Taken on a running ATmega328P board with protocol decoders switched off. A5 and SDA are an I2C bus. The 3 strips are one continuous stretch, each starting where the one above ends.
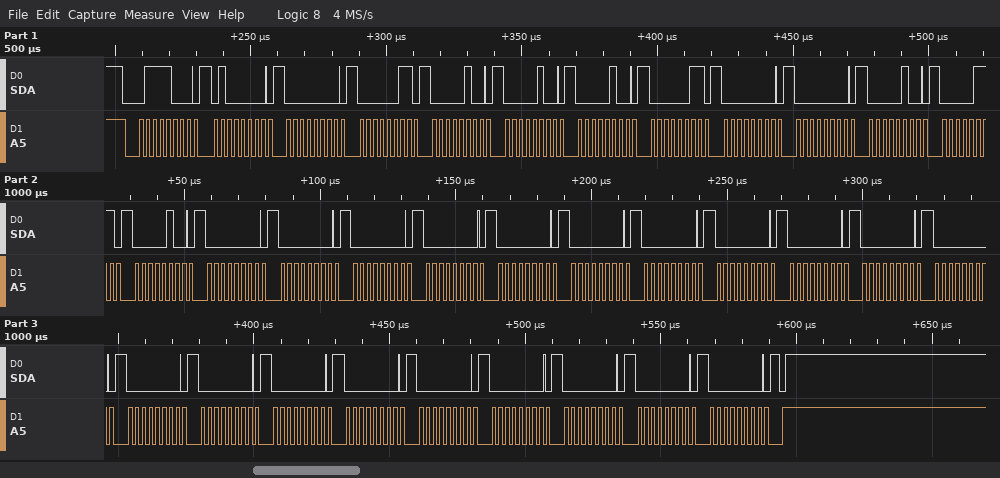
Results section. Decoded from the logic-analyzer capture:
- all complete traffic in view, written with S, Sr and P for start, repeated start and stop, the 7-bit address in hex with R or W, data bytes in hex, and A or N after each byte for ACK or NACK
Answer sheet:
S 3CW A 40 A 00 A 03 A 04 A 04 A 04 A 03 A 00 A 00 A 04 A 07 A 04 A 00 A 00 A 00 A 00 A 00 A 00 A 00 A 00 A 00 A 00 A 00 A 00 A 00 A 00 A 00 A 00 A 00 A 00 A 00 A 00 A P
